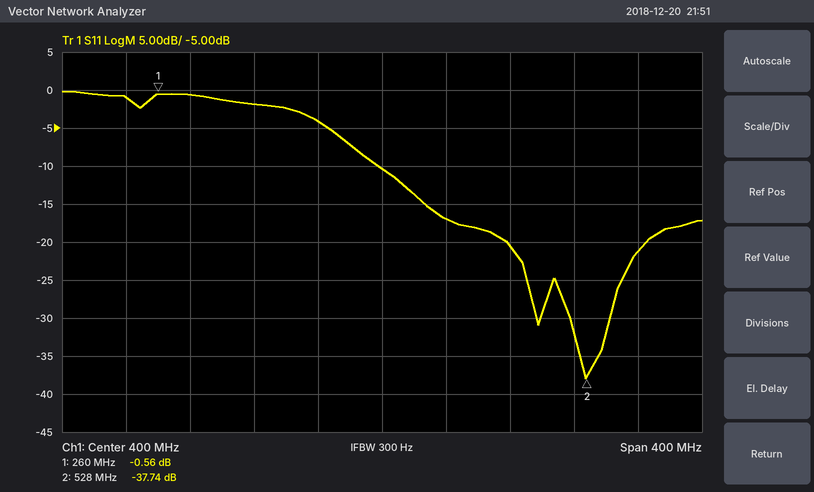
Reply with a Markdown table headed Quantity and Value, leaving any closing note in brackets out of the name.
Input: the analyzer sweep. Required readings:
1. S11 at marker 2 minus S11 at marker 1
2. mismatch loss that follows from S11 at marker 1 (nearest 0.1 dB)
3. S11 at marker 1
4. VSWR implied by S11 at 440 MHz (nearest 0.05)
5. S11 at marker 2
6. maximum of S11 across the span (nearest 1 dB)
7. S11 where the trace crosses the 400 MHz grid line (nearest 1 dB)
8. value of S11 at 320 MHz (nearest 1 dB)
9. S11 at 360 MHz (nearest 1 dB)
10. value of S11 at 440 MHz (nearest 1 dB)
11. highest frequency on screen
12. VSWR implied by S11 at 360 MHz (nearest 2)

| Quantity | Value |
|---|---|
| S11 at marker 2 minus S11 at marker 1 | -37.18 dB |
| mismatch loss that follows from S11 at marker 1 | 9.2 dB |
| S11 at marker 1 | -0.56 dB |
| VSWR implied by S11 at 440 MHz | 1.35 |
| S11 at marker 2 | -37.74 dB |
| maximum of S11 across the span | 0 dB |
| S11 where the trace crosses the 400 MHz grid line | -10 dB |
| value of S11 at 320 MHz | -2 dB |
| S11 at 360 MHz | -4 dB |
| value of S11 at 440 MHz | -17 dB |
| highest frequency on screen | 600 MHz |
| VSWR implied by S11 at 360 MHz | 4 |
